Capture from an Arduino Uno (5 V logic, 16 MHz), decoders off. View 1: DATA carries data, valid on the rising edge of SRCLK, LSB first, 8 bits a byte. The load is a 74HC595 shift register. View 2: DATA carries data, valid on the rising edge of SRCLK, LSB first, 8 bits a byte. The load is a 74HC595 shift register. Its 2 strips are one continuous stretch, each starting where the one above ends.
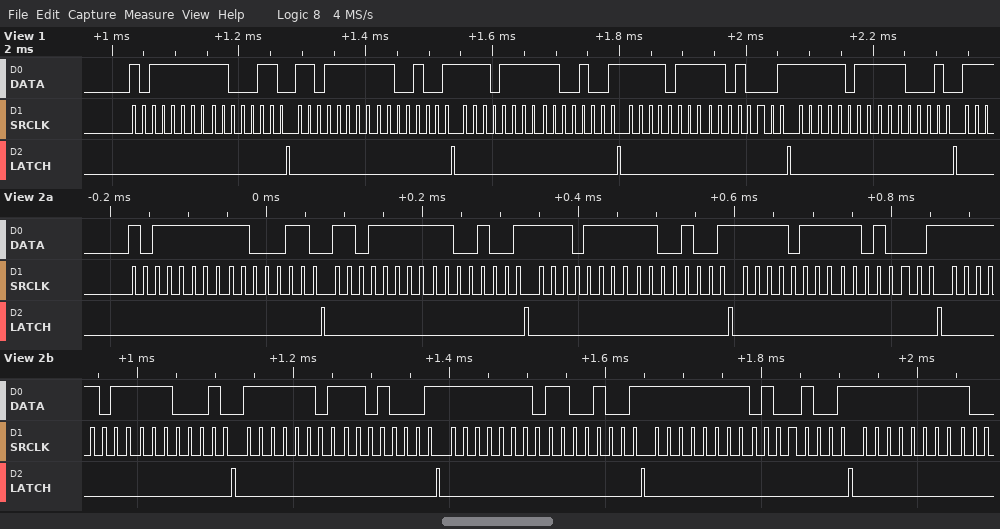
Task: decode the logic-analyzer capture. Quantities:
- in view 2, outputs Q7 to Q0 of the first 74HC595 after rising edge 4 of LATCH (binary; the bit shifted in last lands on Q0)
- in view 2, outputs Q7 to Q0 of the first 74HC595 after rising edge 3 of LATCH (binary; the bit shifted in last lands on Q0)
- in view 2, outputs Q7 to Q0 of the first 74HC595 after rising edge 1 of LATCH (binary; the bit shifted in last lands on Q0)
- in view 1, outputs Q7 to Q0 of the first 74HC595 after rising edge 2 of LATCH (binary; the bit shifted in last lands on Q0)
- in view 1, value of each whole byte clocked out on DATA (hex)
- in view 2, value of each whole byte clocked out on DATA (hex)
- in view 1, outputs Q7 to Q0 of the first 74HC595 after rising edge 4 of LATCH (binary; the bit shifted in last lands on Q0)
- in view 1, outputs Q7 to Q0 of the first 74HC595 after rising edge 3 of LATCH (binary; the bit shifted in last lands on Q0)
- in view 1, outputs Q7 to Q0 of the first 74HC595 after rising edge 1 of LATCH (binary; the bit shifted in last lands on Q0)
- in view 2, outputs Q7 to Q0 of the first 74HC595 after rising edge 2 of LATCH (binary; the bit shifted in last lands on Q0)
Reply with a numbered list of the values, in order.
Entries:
1. 11010001
2. 11001001
3. 11000110
4. 11001001
5. 0xFD 0x63 0xFB 0x93 0xF7 0x93 0xEF 0x8B 0xDF 0x47
6. FD 63 FB 93 F7 93 EF 8B DF 47 BF 8B 7F 93 FF 92 FF
7. 11010001
8. 11001001
9. 11000110
10. 11001001
